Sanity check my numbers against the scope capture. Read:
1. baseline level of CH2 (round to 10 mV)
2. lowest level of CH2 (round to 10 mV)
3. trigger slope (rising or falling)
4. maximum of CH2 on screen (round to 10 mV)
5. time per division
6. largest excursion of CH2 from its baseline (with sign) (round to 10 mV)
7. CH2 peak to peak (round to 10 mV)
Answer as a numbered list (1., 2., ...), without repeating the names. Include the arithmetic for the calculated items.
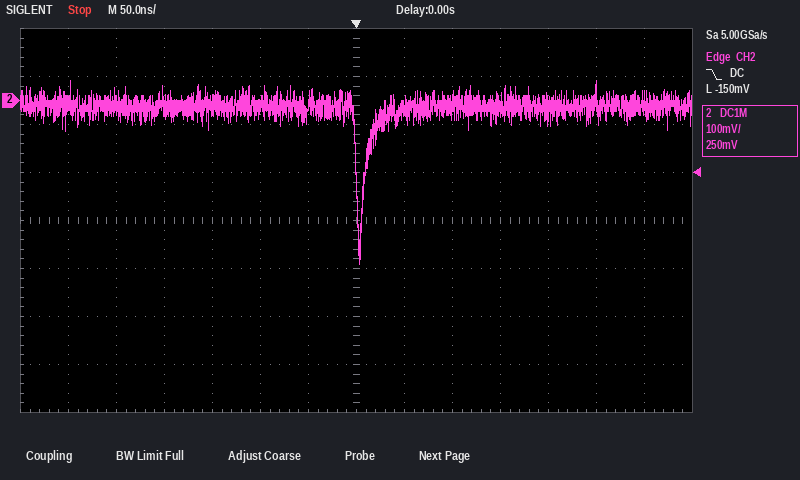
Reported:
1. -10 mV
2. -340 mV
3. falling
4. 40 mV
5. 50 ns
6. -340 mV − (-10 mV) = -330 mV
7. 40 mV − (-340 mV) = 380 mV
